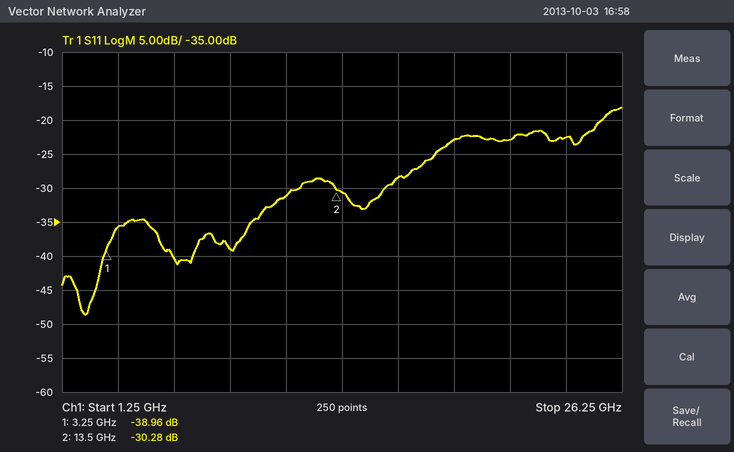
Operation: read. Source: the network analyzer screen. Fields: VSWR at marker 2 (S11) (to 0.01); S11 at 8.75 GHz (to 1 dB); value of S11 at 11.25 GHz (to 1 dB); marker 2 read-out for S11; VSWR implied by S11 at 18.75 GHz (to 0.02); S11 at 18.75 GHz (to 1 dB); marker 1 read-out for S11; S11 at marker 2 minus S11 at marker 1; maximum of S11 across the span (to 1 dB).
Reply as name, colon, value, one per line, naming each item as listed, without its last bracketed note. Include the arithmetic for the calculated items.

VSWR at marker 2 (S11): (1 + 0.0306)/(1 − 0.0306) ≈ 1.06
S11 at 8.75 GHz: -39 dB
value of S11 at 11.25 GHz: -31 dB
marker 2 read-out for S11: -30.28 dB
VSWR implied by S11 at 18.75 GHz: |Γ| = 10^(-23/20) = 0.0708; VSWR = (1 + 0.0708)/(1 − 0.0708) ≈ 1.15, so 1.16 to the nearest 0.02
S11 at 18.75 GHz: -23 dB
marker 1 read-out for S11: -38.96 dB
S11 at marker 2 minus S11 at marker 1: -30.28 − (-38.96) = 8.68 dB
maximum of S11 across the span: -18 dB
